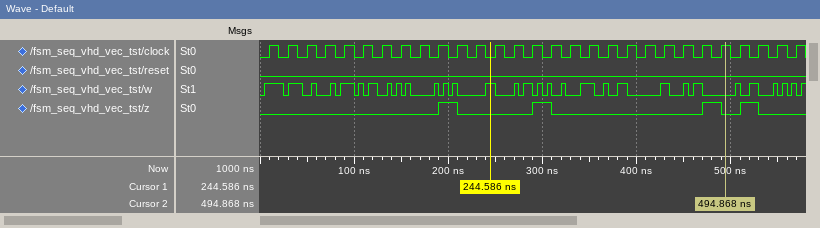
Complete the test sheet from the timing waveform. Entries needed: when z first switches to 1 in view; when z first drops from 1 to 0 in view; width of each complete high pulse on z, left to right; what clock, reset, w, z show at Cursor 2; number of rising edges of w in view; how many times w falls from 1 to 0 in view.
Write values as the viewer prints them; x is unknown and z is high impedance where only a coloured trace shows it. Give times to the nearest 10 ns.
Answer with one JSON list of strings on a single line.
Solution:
["190 ns", "210 ns", "20 ns, 20 ns, 20 ns, 20 ns", "clock=1, reset=0, w=0, z=0", "31", "30"]
